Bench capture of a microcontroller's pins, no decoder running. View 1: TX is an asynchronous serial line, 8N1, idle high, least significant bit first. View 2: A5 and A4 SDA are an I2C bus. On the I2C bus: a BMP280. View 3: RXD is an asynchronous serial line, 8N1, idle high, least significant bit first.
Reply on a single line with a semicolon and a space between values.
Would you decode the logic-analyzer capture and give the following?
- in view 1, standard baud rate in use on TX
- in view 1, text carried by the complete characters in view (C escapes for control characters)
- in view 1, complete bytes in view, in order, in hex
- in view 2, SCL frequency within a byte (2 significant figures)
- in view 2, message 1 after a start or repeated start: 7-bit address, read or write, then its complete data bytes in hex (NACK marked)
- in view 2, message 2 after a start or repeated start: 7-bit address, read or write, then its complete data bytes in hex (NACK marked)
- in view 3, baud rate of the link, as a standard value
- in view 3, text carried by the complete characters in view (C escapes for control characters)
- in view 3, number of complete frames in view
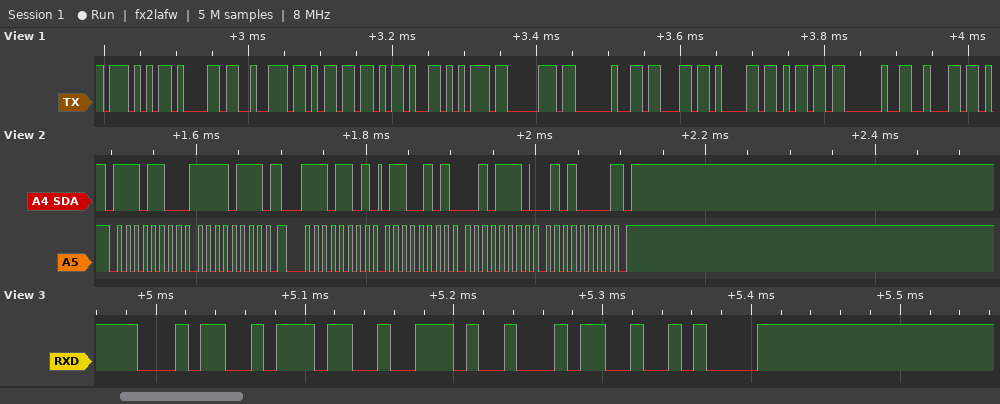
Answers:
115200 baud; "Warm-up cam b"; 0x57 0x61 0x72 0x6D 0x2D 0x75 0x70 0x20 0x63 0x61 0x6D 0x20 0x62; 100 kHz; 0x76 write: F7; 0x76 read: 65 2E 50 NACK; 115200 baud; "47.4\n"; 5
